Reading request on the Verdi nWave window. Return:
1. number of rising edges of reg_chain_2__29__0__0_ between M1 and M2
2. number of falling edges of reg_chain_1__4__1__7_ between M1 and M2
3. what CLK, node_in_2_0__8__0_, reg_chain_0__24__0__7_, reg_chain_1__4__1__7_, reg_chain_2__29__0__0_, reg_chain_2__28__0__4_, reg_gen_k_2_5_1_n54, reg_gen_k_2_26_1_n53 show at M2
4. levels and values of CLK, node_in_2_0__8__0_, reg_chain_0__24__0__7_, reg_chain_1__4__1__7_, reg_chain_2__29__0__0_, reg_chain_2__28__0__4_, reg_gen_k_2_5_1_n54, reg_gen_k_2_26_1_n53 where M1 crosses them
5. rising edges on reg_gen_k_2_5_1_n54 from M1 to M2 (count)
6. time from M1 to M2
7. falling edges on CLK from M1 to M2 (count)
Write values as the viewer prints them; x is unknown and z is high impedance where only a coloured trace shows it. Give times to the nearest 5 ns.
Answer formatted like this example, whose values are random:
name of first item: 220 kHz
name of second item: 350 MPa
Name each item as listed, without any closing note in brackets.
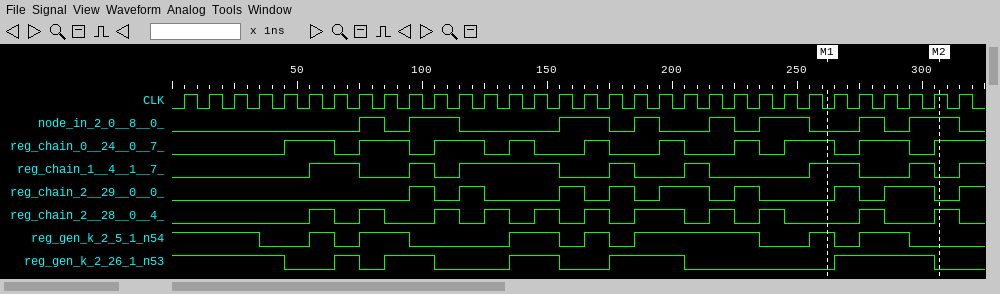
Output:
number of rising edges of reg_chain_2__29__0__0_ between M1 and M2: 2
number of falling edges of reg_chain_1__4__1__7_ between M1 and M2: 2
what CLK, node_in_2_0__8__0_, reg_chain_0__24__0__7_, reg_chain_1__4__1__7_, reg_chain_2__29__0__0_, reg_chain_2__28__0__4_, reg_gen_k_2_5_1_n54, reg_gen_k_2_26_1_n53 show at M2: CLK=1, node_in_2_0__8__0_=1, reg_chain_0__24__0__7_=1, reg_chain_1__4__1__7_=0, reg_chain_2__29__0__0_=0, reg_chain_2__28__0__4_=1, reg_gen_k_2_5_1_n54=0, reg_gen_k_2_26_1_n53=0
levels and values of CLK, node_in_2_0__8__0_, reg_chain_0__24__0__7_, reg_chain_1__4__1__7_, reg_chain_2__29__0__0_, reg_chain_2__28__0__4_, reg_gen_k_2_5_1_n54, reg_gen_k_2_26_1_n53 where M1 crosses them: CLK=0, node_in_2_0__8__0_=0, reg_chain_0__24__0__7_=1, reg_chain_1__4__1__7_=1, reg_chain_2__29__0__0_=0, reg_chain_2__28__0__4_=0, reg_gen_k_2_5_1_n54=1, reg_gen_k_2_26_1_n53=0
rising edges on reg_gen_k_2_5_1_n54 from M1 to M2: 1
time from M1 to M2: 45 ns
falling edges on CLK from M1 to M2: 4
